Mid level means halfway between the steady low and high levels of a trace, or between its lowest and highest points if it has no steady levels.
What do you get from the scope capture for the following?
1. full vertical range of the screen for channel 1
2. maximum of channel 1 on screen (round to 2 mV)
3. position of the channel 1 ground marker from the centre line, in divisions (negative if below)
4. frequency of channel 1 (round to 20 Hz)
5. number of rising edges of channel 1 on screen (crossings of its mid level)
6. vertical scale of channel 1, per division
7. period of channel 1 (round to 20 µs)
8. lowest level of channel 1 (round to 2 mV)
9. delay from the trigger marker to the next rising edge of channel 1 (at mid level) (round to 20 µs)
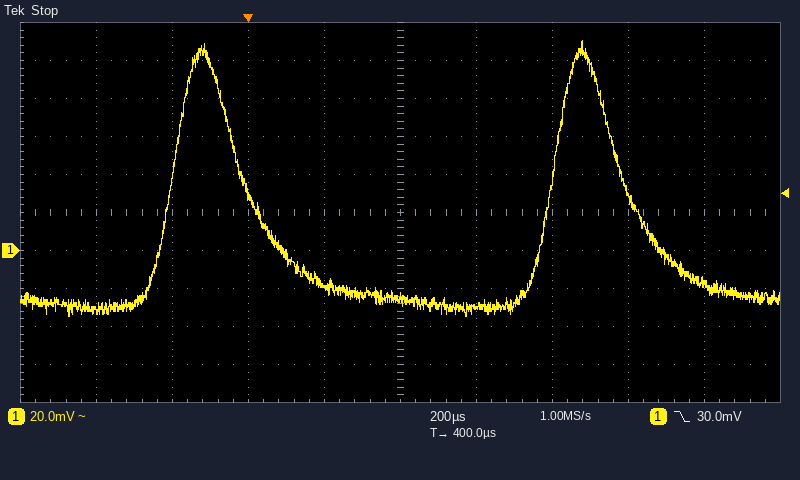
200 mV
110 mV
-1.0 div
1.00 kHz
2
20 mV
1.00 ms
-34 mV
800 µs
